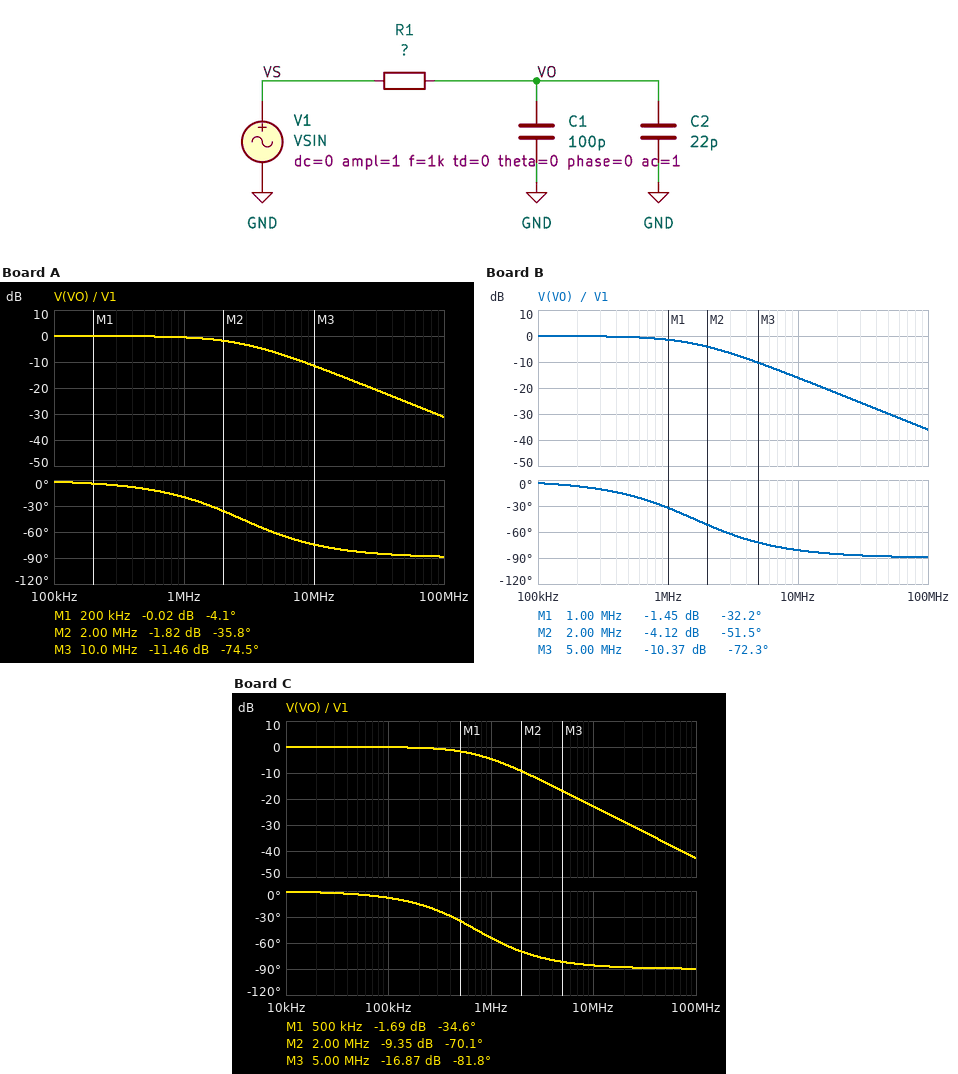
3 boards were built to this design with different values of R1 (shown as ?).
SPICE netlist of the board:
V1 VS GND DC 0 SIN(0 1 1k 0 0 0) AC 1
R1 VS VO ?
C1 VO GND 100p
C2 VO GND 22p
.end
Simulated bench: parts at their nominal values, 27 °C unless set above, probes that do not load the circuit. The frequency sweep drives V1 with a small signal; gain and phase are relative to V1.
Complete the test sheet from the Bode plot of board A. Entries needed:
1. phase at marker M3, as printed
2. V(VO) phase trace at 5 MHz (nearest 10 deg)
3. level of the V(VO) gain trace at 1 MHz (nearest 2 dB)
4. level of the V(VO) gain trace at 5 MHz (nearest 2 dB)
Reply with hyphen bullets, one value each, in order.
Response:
- -74.5 deg
- -60 deg
- 0 dB
- -6 dB
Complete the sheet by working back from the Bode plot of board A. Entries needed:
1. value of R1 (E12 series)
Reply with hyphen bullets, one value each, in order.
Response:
- 470 Ω
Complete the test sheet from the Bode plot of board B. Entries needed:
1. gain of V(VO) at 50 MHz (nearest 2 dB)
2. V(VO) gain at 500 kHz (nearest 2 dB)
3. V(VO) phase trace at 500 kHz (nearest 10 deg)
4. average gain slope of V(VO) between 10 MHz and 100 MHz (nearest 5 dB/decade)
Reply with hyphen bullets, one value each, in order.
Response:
- -30 dB
- 0 dB
- -20 deg
- -20 dB/decade
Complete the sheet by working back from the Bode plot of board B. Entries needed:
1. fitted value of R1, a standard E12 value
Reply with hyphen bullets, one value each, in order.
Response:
- 820 Ω
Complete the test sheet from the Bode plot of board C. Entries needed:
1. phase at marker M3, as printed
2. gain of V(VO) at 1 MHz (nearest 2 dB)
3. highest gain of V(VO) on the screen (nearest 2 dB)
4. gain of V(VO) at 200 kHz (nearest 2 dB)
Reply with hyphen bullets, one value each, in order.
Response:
- -81.8 deg
- -4 dB
- 0 dB
- 0 dB
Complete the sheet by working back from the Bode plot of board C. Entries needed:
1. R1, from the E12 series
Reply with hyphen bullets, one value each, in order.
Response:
- 1.8 kΩ
